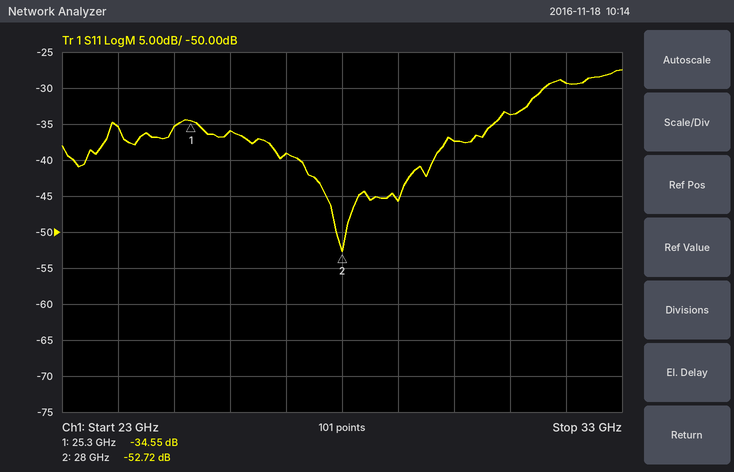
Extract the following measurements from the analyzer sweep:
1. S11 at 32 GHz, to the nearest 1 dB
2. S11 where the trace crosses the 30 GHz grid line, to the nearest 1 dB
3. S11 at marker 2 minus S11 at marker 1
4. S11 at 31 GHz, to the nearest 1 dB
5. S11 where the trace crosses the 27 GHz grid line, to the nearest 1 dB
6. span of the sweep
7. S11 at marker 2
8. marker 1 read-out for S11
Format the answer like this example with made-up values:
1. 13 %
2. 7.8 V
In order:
1. -29 dB
2. -37 dB
3. -18.17 dB
4. -34 dB
5. -39 dB
6. 10 GHz
7. -52.72 dB
8. -34.55 dB
